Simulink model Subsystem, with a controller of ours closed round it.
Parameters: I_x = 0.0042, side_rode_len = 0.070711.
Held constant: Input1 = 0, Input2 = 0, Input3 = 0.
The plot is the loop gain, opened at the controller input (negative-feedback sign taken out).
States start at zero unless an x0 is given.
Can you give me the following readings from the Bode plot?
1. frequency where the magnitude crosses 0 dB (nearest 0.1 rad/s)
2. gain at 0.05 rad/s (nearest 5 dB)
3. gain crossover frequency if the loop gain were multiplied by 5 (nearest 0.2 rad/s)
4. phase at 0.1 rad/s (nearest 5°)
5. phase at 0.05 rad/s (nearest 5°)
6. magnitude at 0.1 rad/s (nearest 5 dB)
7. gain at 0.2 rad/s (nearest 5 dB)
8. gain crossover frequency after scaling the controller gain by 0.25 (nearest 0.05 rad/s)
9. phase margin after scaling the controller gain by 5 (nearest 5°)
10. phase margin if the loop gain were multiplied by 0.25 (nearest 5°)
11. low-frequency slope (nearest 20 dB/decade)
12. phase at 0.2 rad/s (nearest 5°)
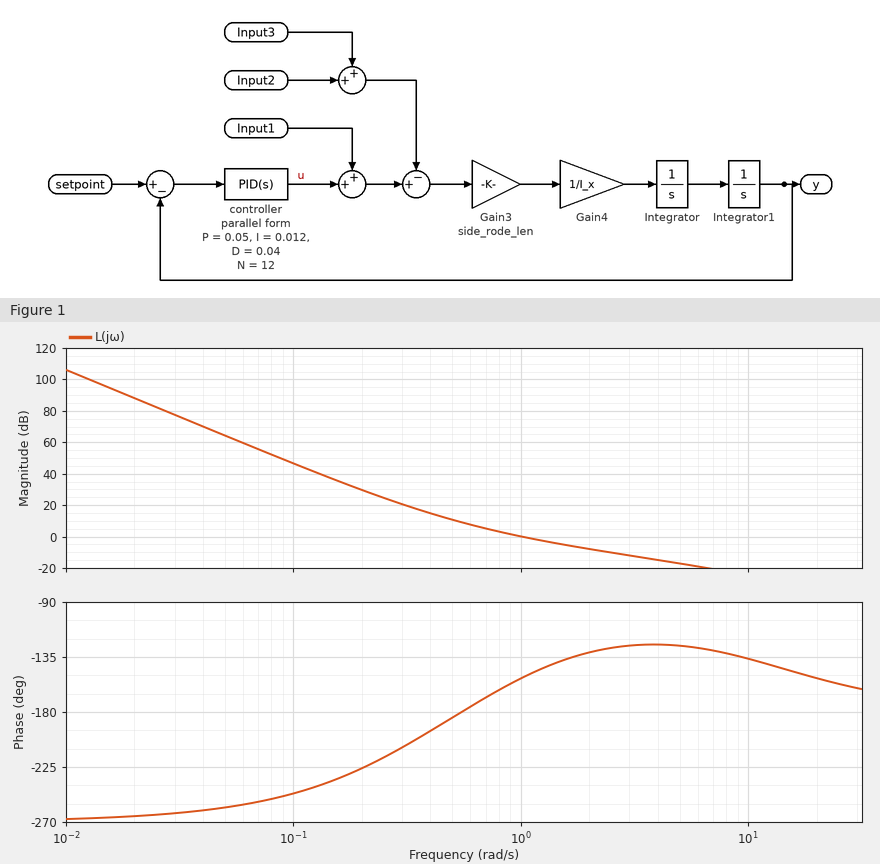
1.0 rad/s
65 dB
3.6 rad/s
-245°
-260°
45 dB
30 dB
0.45 rad/s
55°
-10°
-60 dB/decade
-225°
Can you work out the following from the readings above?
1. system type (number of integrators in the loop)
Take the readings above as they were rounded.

3
